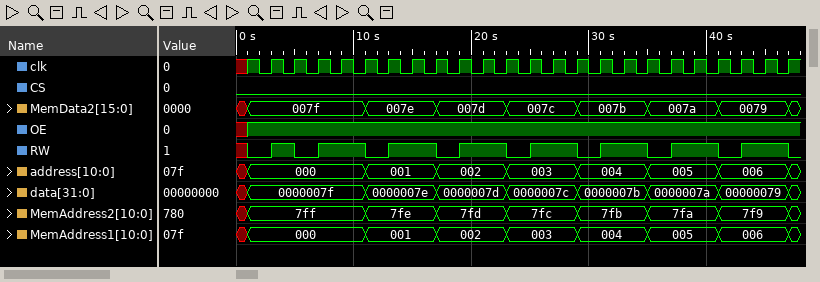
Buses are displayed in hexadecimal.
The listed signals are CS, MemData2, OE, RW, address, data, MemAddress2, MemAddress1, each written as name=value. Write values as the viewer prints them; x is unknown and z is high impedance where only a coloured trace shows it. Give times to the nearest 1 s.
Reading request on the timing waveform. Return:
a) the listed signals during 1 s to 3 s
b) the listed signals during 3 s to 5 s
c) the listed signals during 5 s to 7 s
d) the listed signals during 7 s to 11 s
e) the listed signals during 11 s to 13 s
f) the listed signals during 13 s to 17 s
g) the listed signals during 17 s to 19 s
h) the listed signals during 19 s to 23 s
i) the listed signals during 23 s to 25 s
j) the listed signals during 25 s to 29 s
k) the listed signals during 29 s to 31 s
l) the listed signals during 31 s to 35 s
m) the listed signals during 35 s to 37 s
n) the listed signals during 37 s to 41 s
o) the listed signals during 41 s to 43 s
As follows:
CS=0, MemData2=007f, OE=1, RW=0, address=000, data=0000007f, MemAddress2=7ff, MemAddress1=000
CS=0, MemData2=007f, OE=1, RW=1, address=000, data=0000007f, MemAddress2=7ff, MemAddress1=000
CS=0, MemData2=007f, OE=1, RW=0, address=000, data=0000007f, MemAddress2=7ff, MemAddress1=000
CS=0, MemData2=007f, OE=1, RW=1, address=000, data=0000007f, MemAddress2=7ff, MemAddress1=000
CS=0, MemData2=007e, OE=1, RW=0, address=001, data=0000007e, MemAddress2=7fe, MemAddress1=001
CS=0, MemData2=007e, OE=1, RW=1, address=001, data=0000007e, MemAddress2=7fe, MemAddress1=001
CS=0, MemData2=007d, OE=1, RW=0, address=002, data=0000007d, MemAddress2=7fd, MemAddress1=002
CS=0, MemData2=007d, OE=1, RW=1, address=002, data=0000007d, MemAddress2=7fd, MemAddress1=002
CS=0, MemData2=007c, OE=1, RW=0, address=003, data=0000007c, MemAddress2=7fc, MemAddress1=003
CS=0, MemData2=007c, OE=1, RW=1, address=003, data=0000007c, MemAddress2=7fc, MemAddress1=003
CS=0, MemData2=007b, OE=1, RW=0, address=004, data=0000007b, MemAddress2=7fb, MemAddress1=004
CS=0, MemData2=007b, OE=1, RW=1, address=004, data=0000007b, MemAddress2=7fb, MemAddress1=004
CS=0, MemData2=007a, OE=1, RW=0, address=005, data=0000007a, MemAddress2=7fa, MemAddress1=005
CS=0, MemData2=007a, OE=1, RW=1, address=005, data=0000007a, MemAddress2=7fa, MemAddress1=005
CS=0, MemData2=0079, OE=1, RW=0, address=006, data=00000079, MemAddress2=7f9, MemAddress1=006
